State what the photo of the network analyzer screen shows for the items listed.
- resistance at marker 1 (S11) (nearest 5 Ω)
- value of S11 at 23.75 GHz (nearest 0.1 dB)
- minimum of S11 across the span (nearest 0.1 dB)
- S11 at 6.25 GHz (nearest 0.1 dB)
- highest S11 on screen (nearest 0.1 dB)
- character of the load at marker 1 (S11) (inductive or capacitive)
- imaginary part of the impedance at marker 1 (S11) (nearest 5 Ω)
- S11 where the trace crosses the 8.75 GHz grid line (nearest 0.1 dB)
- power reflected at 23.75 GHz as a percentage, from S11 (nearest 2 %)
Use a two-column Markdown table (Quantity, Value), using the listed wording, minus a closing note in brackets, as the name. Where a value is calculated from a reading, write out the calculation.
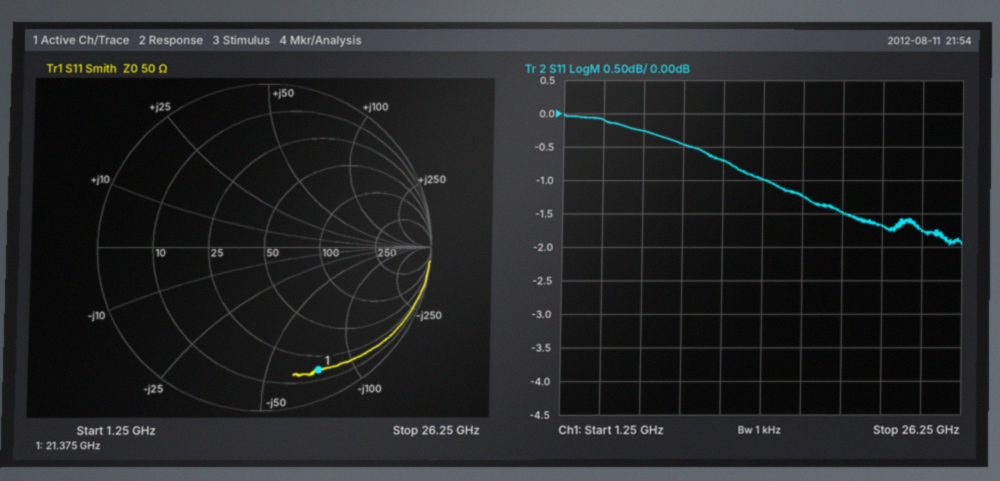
| Quantity | Value |
|---|---|
| resistance at marker 1 (S11) | 15 Ω |
| value of S11 at 23.75 GHz | -1.8 dB |
| minimum of S11 across the span | -2.0 dB |
| S11 at 6.25 GHz | -0.3 dB |
| highest S11 on screen | 0.0 dB |
| character of the load at marker 1 (S11) | capacitive |
| imaginary part of the impedance at marker 1 (S11) | -75 Ω |
| S11 where the trace crosses the 8.75 GHz grid line | -0.5 dB |
| power reflected at 23.75 GHz as a percentage, from S11 | 10^(-1.8/10) ≈ 66 % |
